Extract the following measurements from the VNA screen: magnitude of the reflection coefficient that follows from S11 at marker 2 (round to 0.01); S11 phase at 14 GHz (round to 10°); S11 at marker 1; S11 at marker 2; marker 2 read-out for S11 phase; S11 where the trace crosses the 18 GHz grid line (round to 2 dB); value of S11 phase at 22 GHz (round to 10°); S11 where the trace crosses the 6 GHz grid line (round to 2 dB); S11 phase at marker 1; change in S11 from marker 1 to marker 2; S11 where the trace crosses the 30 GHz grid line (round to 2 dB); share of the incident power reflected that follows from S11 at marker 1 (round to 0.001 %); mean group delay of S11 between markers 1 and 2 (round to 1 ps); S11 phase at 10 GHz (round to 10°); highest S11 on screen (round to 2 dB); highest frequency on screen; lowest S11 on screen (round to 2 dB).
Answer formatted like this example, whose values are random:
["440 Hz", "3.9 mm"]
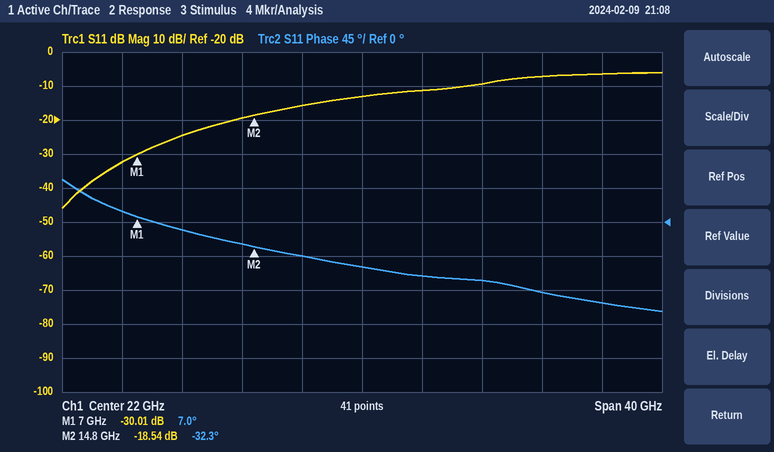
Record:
["0.12", "-30°", "-30.01 dB", "-18.54 dB", "-32.3°", "-16 dB", "-60°", "-32 dB", "7.0°", "11.47 dB", "-10 dB", "0.100 %", "14 ps", "-10°", "-6 dB", "42 GHz", "-46 dB"]
